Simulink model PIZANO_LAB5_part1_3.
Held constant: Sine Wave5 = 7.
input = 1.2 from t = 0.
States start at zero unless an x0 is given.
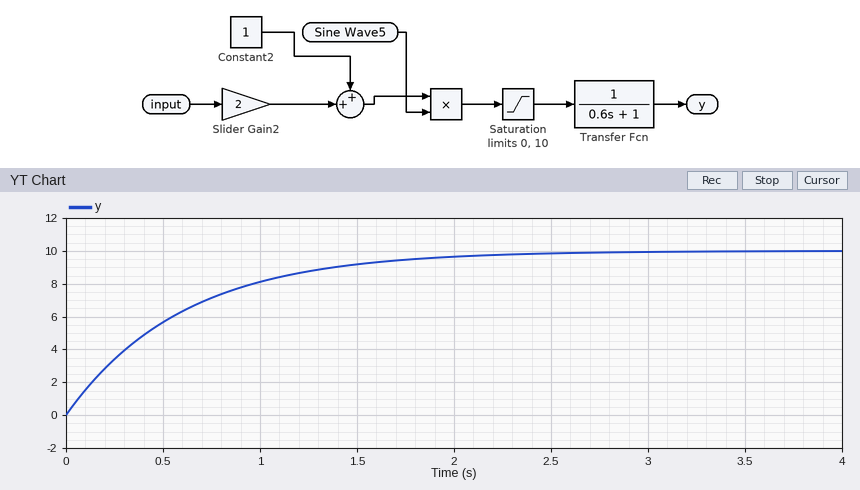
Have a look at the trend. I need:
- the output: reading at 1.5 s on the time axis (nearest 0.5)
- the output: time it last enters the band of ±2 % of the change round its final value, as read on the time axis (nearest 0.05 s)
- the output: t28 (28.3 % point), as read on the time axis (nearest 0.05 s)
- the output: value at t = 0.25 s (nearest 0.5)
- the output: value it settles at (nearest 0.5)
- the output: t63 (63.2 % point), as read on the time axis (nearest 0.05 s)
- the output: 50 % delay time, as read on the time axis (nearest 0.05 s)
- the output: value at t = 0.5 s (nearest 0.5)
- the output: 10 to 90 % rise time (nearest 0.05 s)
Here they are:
9.0
2.35 s
0.20 s
3.5
10.0
0.60 s
0.40 s
5.5
1.30 s
